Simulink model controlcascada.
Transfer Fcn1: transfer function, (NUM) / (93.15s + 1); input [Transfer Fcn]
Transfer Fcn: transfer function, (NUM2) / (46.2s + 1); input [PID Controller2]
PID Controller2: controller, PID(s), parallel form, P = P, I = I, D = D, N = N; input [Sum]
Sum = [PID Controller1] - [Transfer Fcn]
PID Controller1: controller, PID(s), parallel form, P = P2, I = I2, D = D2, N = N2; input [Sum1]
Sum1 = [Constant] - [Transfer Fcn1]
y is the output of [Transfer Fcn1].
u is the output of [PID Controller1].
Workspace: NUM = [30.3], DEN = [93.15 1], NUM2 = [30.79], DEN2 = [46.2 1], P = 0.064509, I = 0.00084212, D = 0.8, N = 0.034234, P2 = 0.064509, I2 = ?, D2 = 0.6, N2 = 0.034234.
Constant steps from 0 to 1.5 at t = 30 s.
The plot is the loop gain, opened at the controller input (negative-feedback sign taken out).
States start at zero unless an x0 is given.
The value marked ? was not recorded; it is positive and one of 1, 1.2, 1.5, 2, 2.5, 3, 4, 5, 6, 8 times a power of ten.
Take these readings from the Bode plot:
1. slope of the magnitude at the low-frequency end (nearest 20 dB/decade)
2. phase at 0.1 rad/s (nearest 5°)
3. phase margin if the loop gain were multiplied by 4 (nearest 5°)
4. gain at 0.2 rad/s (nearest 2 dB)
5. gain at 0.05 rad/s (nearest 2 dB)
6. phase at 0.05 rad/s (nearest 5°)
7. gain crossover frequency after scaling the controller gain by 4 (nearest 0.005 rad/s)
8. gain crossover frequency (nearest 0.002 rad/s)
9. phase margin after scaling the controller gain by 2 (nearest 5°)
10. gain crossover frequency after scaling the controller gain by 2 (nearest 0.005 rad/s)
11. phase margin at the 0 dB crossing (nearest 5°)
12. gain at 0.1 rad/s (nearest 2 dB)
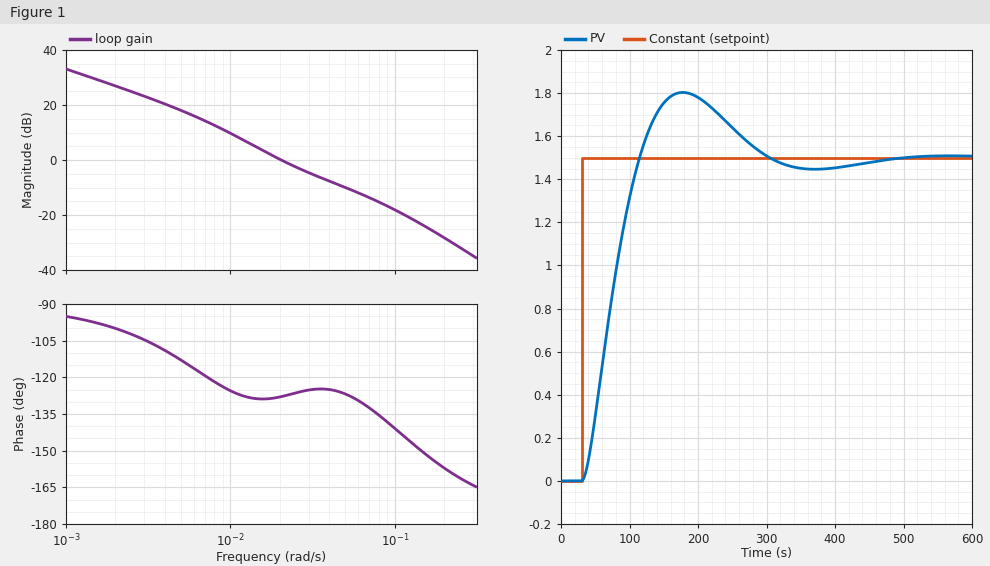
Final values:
-20 dB/decade
-140°
50°
-28 dB
-10 dB
-125°
0.060 rad/s
0.020 rad/s
55°
0.035 rad/s
50°
-18 dB
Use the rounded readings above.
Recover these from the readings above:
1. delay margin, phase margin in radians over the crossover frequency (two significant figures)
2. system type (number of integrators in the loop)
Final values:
44 s
1
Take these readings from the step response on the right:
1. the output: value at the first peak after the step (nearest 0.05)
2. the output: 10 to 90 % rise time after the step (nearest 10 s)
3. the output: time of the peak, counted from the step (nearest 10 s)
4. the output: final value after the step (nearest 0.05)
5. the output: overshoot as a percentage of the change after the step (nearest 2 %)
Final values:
1.80
60 s
150 s
1.50
20 %
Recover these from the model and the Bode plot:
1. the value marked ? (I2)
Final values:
0.0015
